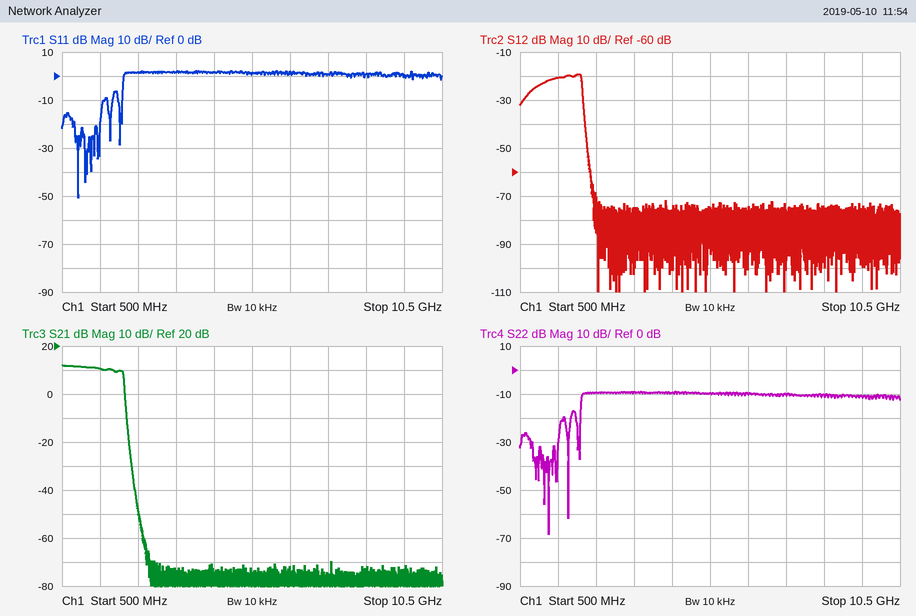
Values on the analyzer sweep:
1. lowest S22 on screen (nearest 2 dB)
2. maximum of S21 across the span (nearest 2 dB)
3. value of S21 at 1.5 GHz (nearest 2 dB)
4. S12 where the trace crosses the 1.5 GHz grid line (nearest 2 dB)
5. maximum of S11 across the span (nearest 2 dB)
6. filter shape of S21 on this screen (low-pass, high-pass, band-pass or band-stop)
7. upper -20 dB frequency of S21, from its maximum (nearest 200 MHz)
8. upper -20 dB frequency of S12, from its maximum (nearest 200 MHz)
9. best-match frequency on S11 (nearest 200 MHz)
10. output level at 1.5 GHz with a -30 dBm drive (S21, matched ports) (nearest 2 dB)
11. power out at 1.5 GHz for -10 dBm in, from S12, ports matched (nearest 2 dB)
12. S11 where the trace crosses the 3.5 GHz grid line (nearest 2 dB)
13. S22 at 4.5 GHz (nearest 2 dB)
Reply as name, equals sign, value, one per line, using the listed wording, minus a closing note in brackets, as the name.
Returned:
lowest S22 on screen = -68 dB
maximum of S21 across the span = 12 dB
value of S21 at 1.5 GHz = 10 dB
S12 where the trace crosses the 1.5 GHz grid line = -20 dB
maximum of S11 across the span = 2 dB
filter shape of S21 on this screen = low-pass
upper -20 dB frequency of S21, from its maximum = 2.2 GHz
upper -20 dB frequency of S12, from its maximum = 2.2 GHz
best-match frequency on S11 = 1.0 GHz
output level at 1.5 GHz with a -30 dBm drive (S21, matched ports) = -20 dBm
power out at 1.5 GHz for -10 dBm in, from S12, ports matched = -30 dBm
S11 where the trace crosses the 3.5 GHz grid line = 2 dB
S22 at 4.5 GHz = -10 dB
